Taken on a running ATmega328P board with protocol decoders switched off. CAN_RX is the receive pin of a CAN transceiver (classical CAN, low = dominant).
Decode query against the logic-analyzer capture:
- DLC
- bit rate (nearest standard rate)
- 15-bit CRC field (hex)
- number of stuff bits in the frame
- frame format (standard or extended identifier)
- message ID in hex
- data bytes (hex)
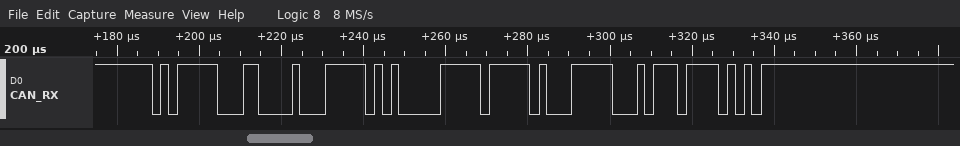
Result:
4
500 kbit/s
0x177A
6
standard
0x5F3
7E 83 FF 1F
